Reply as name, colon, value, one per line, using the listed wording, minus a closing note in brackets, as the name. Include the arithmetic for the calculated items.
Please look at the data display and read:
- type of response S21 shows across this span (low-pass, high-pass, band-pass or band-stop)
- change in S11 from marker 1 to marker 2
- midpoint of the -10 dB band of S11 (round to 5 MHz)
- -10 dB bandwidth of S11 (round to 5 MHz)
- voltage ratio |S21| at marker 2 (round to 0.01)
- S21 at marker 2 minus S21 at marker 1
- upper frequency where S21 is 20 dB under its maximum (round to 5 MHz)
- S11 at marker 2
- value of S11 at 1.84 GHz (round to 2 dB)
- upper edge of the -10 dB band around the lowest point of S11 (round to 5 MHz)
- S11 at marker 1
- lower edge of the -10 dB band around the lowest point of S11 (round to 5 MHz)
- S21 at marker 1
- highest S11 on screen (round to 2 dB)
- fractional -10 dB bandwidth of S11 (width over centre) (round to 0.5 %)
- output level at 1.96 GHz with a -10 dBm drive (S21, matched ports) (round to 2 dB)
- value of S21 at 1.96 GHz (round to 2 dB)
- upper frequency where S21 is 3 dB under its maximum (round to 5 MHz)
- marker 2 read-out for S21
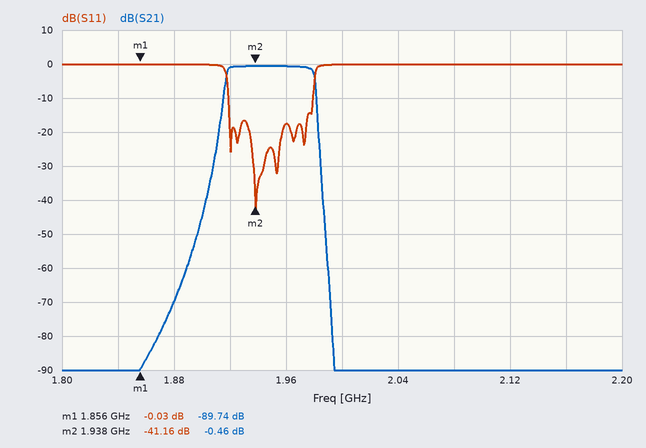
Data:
type of response S21 shows across this span: band-pass
change in S11 from marker 1 to marker 2: -41.16 − (-0.03) = -41.13 dB
midpoint of the -10 dB band of S11: 1.950 GHz
-10 dB bandwidth of S11: 1.980 GHz − 1.920 GHz = 60 MHz
voltage ratio |S21| at marker 2: 10^(-0.46/20) ≈ 0.95
S21 at marker 2 minus S21 at marker 1: -0.46 − (-89.74) = 89.28 dB
upper frequency where S21 is 20 dB under its maximum: 1.985 GHz
S11 at marker 2: -41.16 dB
value of S11 at 1.84 GHz: 0 dB
upper edge of the -10 dB band around the lowest point of S11: 1.980 GHz
S11 at marker 1: -0.03 dB
lower edge of the -10 dB band around the lowest point of S11: 1.920 GHz
S21 at marker 1: -89.74 dB
highest S11 on screen: 0 dB
fractional -10 dB bandwidth of S11 (width over centre): 60 MHz / 1.95 GHz ≈ 3.08 %, so 3.0 % to the nearest 0.5 %
output level at 1.96 GHz with a -10 dBm drive (S21, matched ports): -10 dBm + (0 dB) = -10 dBm
value of S21 at 1.96 GHz: 0 dB
upper frequency where S21 is 3 dB under its maximum: 1.980 GHz
marker 2 read-out for S21: -0.46 dB
